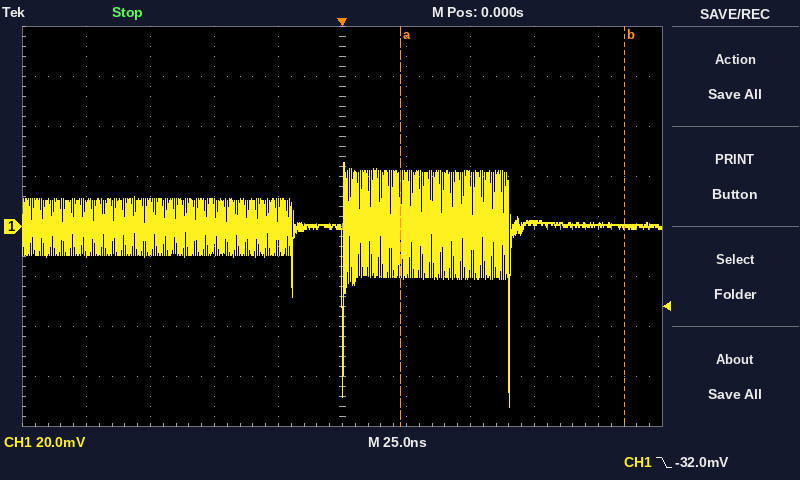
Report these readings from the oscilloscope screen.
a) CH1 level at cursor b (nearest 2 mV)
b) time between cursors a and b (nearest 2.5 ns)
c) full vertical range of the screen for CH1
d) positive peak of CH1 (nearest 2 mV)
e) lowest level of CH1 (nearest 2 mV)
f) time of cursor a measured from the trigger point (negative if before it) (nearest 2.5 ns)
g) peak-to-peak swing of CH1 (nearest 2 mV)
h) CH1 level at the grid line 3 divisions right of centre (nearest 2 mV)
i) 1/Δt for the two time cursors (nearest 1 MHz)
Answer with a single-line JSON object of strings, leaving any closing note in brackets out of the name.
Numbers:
{"CH1 level at cursor b": "0 mV", "time between cursors a and b": "87.5 ns", "full vertical range of the screen for CH1": "160 mV", "positive peak of CH1": "26 mV", "lowest level of CH1": "-72 mV", "time of cursor a measured from the trigger point (negative if before it)": "+22.5 ns", "peak-to-peak swing of CH1": "98 mV", "CH1 level at the grid line 3 divisions right of centre": "2 mV", "1/Δt for the two time cursors": "11 MHz"}
